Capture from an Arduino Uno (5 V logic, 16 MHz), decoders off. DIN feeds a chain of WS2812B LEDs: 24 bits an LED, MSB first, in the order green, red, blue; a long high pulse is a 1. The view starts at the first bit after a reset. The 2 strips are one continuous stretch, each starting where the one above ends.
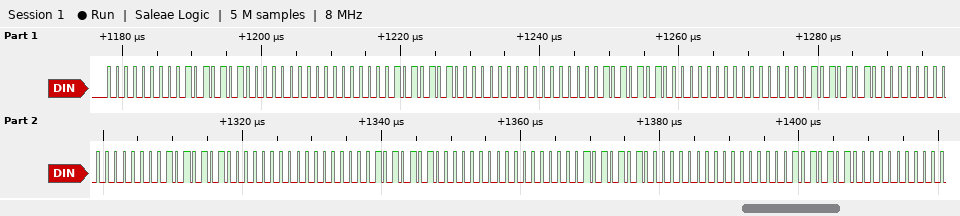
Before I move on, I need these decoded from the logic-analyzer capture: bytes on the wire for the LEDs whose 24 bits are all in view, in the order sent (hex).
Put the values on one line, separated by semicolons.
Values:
00 55 00 00 55 00 00 55 00 00 55 00 00 55 00 00 55 00 00 55 00 00 55 00
